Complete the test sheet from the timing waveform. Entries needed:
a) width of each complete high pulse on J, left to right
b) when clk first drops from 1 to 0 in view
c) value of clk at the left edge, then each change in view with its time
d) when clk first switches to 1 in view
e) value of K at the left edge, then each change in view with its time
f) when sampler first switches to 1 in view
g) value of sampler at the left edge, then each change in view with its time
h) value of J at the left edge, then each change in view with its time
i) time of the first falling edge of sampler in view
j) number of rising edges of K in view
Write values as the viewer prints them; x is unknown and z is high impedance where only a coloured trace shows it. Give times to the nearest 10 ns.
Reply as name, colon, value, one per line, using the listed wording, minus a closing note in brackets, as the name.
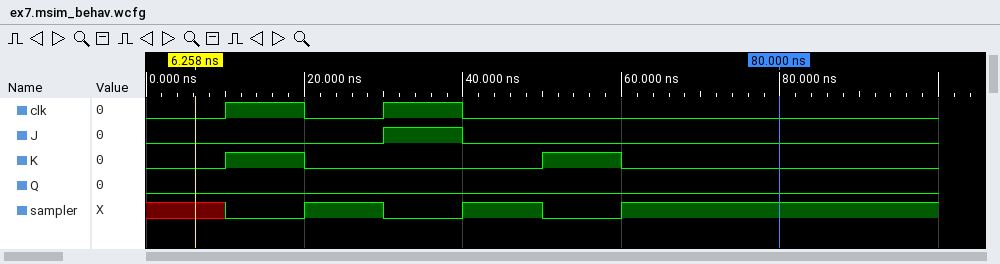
width of each complete high pulse on J, left to right: 10 ns
when clk first drops from 1 to 0 in view: 20 ns
value of clk at the left edge, then each change in view with its time: 0, 1 at 10 ns, 0 at 20 ns, 1 at 30 ns, 0 at 40 ns
when clk first switches to 1 in view: 10 ns
value of K at the left edge, then each change in view with its time: 0, 1 at 10 ns, 0 at 20 ns, 1 at 50 ns, 0 at 60 ns
when sampler first switches to 1 in view: 20 ns
value of sampler at the left edge, then each change in view with its time: x, 0 at 10 ns, 1 at 20 ns, 0 at 30 ns, 1 at 40 ns, 0 at 50 ns, 1 at 60 ns
value of J at the left edge, then each change in view with its time: 0, 1 at 30 ns, 0 at 40 ns
time of the first falling edge of sampler in view: 30 ns
number of rising edges of K in view: 2
